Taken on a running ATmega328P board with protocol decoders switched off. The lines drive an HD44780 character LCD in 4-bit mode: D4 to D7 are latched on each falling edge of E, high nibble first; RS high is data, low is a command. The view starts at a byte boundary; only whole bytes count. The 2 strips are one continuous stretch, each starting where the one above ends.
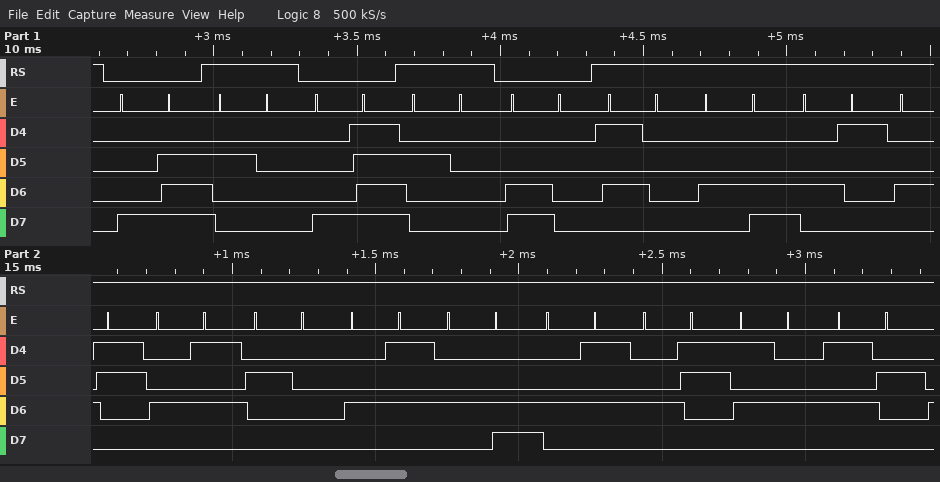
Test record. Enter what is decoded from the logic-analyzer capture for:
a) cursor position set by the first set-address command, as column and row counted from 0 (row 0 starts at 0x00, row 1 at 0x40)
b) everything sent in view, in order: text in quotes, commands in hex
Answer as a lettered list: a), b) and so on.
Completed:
a) column 14, row 0
b) 0x8E " " 0x8F " " 0xC0 "PLACE ELECTR"
